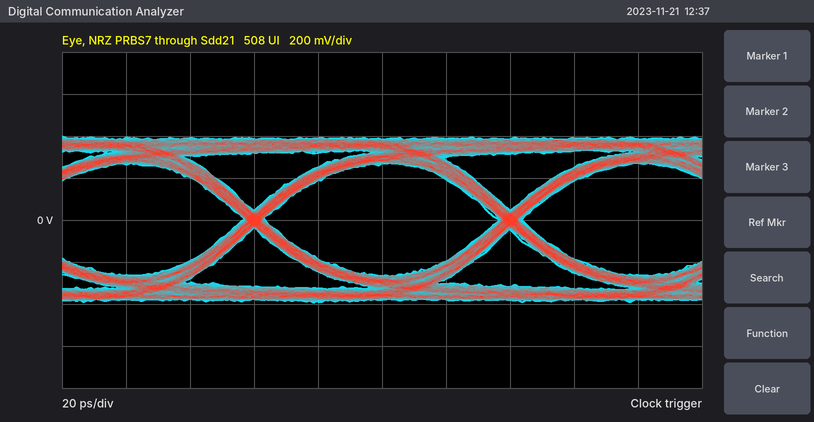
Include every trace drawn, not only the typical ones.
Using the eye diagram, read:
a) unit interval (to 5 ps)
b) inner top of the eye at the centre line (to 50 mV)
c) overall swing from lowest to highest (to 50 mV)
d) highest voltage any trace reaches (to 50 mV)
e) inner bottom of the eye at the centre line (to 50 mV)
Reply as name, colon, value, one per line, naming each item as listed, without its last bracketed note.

unit interval: 80 ps
inner top of the eye at the centre line: 250 mV
overall swing from lowest to highest: 800 mV
highest voltage any trace reaches: 400 mV
inner bottom of the eye at the centre line: -250 mV
